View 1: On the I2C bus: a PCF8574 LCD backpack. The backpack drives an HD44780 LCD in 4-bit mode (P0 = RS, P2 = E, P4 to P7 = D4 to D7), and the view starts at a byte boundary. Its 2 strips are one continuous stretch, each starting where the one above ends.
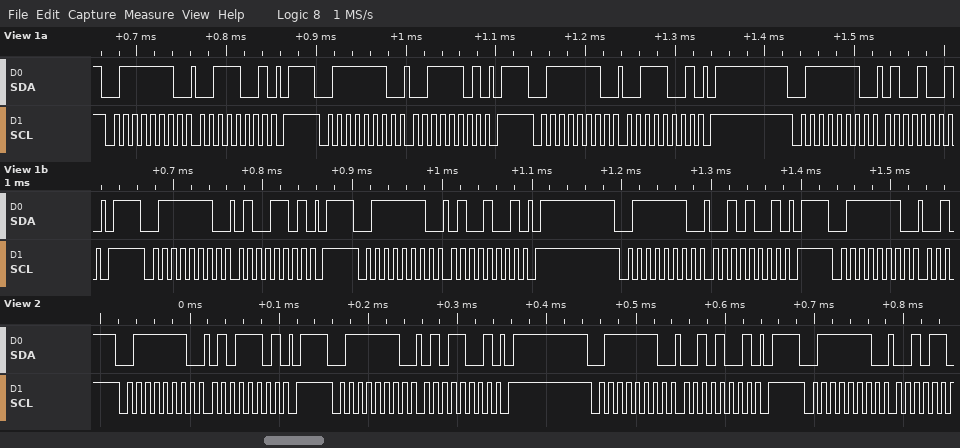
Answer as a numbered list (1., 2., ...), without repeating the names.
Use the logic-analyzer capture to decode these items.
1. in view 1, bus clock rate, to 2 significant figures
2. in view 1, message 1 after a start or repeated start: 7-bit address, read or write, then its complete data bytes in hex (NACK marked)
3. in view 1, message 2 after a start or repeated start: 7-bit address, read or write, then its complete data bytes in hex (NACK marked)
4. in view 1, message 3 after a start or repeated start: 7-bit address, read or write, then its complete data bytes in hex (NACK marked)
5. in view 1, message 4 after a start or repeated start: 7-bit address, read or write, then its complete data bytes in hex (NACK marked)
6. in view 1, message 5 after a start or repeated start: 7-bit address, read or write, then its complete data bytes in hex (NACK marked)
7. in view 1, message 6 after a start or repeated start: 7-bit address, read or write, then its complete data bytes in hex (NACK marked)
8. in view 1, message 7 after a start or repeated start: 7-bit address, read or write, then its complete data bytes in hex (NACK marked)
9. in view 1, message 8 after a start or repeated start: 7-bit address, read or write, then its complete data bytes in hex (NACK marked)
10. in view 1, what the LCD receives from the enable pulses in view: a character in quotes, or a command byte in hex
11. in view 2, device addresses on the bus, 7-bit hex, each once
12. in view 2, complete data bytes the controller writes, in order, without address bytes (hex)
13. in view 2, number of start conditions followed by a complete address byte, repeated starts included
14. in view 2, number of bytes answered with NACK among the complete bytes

1. 100 kHz
2. 0x3F write: 39
3. 0x3F write: 3D
4. 0x3F write: 39
5. 0x3F write: 49
6. 0x3F write: 4D
7. 0x3F write: 49
8. 0x3F write: 29
9. 0x3F write
10. '4'
11. 0x3F
12. 5D 59 29
13. 4
14. 0
